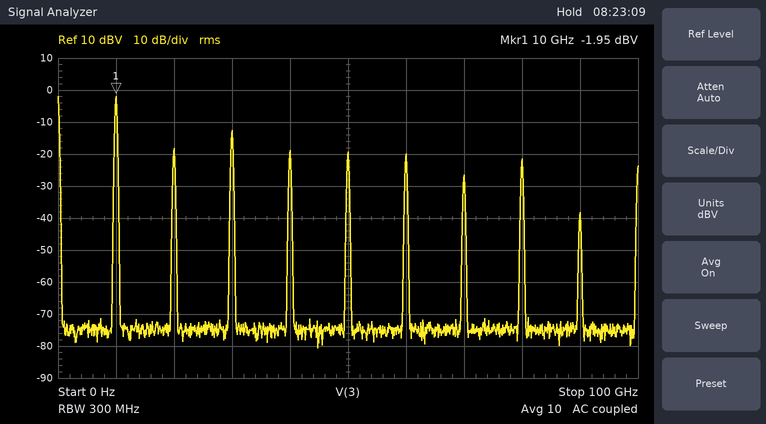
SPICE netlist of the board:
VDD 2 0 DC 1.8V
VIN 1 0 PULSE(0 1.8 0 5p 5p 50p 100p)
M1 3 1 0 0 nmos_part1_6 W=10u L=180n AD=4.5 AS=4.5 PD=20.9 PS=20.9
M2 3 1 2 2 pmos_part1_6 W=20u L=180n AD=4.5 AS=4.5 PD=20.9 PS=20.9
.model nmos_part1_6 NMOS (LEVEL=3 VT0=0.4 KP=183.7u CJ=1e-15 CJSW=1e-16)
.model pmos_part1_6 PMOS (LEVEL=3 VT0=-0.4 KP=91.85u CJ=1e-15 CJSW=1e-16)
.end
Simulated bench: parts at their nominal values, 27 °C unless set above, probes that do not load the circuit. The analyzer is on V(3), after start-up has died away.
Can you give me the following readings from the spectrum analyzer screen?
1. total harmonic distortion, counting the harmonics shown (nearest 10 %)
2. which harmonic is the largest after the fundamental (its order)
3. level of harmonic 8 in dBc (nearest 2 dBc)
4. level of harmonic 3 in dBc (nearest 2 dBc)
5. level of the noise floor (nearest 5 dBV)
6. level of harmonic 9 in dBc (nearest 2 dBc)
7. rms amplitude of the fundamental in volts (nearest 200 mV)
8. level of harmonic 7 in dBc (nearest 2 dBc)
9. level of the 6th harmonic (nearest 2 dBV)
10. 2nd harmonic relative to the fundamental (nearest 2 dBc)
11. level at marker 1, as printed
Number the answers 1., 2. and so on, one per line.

1. 40 %
2. 3
3. -20 dBc
4. -10 dBc
5. -75 dBV
6. -36 dBc
7. 800 mV
8. -24 dBc
9. -20 dBV
10. -16 dBc
11. -1.95 dBV
